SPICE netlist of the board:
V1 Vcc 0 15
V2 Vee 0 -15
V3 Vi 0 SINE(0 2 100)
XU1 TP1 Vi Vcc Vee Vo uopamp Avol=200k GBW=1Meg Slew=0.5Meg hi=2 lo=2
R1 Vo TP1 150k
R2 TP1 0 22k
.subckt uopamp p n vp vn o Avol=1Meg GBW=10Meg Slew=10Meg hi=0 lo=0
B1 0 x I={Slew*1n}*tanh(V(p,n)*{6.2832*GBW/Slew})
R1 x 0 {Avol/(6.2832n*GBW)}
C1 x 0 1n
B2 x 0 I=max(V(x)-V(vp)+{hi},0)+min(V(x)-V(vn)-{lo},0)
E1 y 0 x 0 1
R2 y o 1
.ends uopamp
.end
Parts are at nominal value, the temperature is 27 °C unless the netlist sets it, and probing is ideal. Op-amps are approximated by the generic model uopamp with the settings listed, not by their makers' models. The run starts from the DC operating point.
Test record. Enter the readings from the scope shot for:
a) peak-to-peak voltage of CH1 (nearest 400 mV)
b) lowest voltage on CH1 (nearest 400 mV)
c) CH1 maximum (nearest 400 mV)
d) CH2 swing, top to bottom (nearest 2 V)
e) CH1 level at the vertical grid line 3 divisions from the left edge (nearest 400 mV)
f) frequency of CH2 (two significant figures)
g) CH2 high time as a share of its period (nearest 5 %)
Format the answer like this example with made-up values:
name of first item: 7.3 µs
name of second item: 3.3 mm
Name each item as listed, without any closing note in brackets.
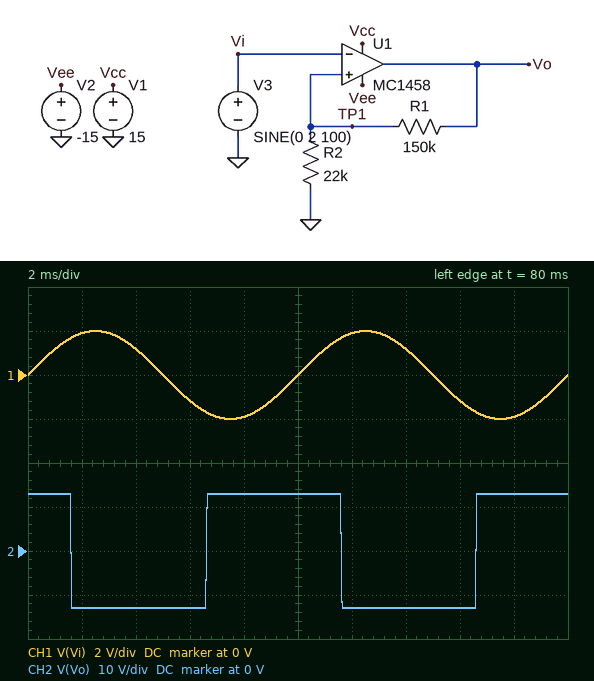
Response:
peak-to-peak voltage of CH1: 4.0 V
lowest voltage on CH1: -2.0 V
CH1 maximum: 2.0 V
CH2 swing, top to bottom: 26 V
CH1 level at the vertical grid line 3 divisions from the left edge: -1.2 V
frequency of CH2: 100 Hz
CH2 high time as a share of its period: 50 %
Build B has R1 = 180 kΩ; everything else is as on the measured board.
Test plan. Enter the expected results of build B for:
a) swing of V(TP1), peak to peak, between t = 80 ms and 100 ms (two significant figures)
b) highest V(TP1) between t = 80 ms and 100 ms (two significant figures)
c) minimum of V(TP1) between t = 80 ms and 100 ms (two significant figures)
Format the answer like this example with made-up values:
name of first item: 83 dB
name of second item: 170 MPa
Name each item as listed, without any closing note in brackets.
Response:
swing of V(TP1), peak to peak, between t = 80 ms and 100 ms: 2.8 V
highest V(TP1) between t = 80 ms and 100 ms: 1.4 V
minimum of V(TP1) between t = 80 ms and 100 ms: -1.4 V
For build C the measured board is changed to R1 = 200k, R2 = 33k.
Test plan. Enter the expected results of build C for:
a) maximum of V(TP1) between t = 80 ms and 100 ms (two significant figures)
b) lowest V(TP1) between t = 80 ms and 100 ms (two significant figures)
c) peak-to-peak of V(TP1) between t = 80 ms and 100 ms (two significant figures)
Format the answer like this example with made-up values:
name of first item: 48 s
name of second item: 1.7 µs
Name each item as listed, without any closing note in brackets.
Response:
maximum of V(TP1) between t = 80 ms and 100 ms: 1.8 V
lowest V(TP1) between t = 80 ms and 100 ms: -1.8 V
peak-to-peak of V(TP1) between t = 80 ms and 100 ms: 3.7 V
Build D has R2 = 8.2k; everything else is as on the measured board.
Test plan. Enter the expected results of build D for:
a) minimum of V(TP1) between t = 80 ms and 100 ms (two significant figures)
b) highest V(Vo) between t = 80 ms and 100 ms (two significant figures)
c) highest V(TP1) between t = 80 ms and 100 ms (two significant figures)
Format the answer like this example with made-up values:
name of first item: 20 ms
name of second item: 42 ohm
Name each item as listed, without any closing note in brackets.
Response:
minimum of V(TP1) between t = 80 ms and 100 ms: -670 mV
highest V(Vo) between t = 80 ms and 100 ms: 13 V
highest V(TP1) between t = 80 ms and 100 ms: 670 mV
